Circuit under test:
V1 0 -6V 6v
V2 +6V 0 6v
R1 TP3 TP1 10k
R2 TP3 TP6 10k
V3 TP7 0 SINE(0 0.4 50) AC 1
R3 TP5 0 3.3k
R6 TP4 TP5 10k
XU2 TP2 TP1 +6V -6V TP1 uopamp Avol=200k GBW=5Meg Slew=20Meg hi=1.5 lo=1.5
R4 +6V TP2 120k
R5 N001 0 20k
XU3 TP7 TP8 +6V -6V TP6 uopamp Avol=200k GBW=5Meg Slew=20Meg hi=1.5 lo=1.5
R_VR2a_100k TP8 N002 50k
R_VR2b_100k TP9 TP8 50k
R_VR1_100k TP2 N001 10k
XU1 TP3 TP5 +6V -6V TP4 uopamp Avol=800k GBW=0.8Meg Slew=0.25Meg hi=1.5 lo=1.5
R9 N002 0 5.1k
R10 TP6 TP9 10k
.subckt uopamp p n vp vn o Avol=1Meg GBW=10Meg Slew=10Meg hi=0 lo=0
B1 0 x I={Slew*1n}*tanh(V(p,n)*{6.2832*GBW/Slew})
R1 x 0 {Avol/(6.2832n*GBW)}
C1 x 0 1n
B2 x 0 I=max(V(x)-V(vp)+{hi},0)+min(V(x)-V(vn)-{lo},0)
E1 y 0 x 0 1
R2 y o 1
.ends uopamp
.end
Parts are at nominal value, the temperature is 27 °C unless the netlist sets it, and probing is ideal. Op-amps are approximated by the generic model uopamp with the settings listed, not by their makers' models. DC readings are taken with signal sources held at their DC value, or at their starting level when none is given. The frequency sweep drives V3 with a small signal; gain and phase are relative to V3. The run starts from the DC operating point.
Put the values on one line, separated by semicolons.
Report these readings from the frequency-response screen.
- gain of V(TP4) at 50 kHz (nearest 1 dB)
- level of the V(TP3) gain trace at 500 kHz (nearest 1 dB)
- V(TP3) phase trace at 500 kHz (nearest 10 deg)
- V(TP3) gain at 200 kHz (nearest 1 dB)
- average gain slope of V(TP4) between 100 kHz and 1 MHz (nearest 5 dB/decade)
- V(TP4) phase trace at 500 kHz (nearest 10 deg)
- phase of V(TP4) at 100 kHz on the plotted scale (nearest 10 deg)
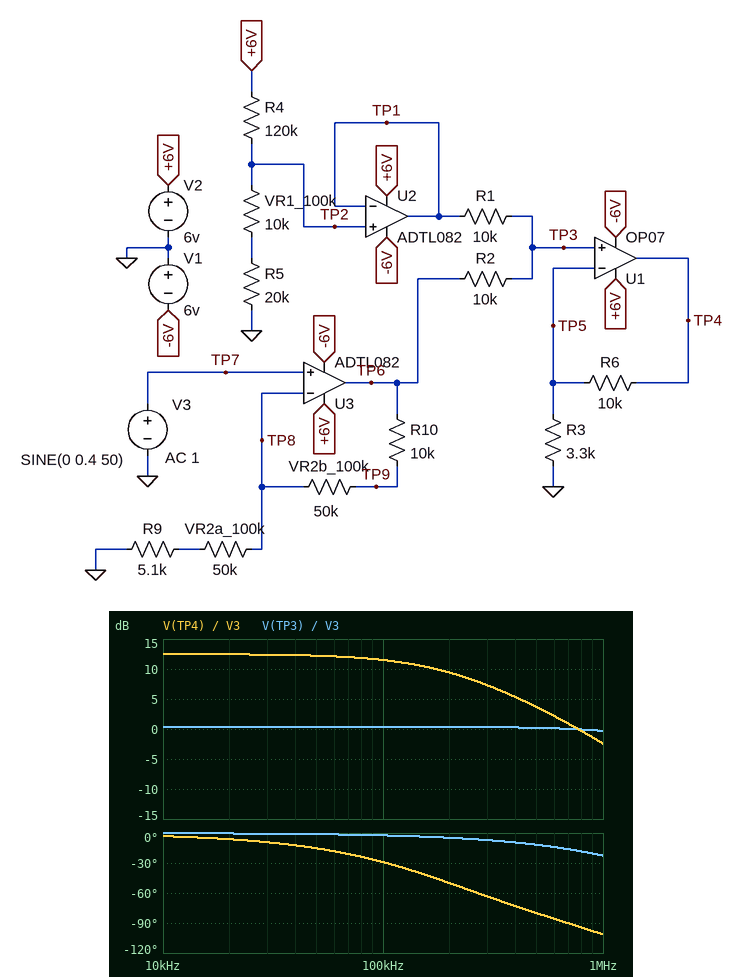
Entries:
12 dB; 0 dB; -10 deg; 0 dB; -15 dB/decade; -80 deg; -30 deg
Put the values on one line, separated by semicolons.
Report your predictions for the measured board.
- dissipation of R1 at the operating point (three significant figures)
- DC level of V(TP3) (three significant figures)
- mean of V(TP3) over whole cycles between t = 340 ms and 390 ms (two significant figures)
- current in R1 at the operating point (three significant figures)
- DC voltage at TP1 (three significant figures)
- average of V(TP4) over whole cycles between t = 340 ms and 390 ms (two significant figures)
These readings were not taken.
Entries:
36.0 µW; 600 mV; 600 mV; 60.0 µA; 1.20 V; 2.4 V
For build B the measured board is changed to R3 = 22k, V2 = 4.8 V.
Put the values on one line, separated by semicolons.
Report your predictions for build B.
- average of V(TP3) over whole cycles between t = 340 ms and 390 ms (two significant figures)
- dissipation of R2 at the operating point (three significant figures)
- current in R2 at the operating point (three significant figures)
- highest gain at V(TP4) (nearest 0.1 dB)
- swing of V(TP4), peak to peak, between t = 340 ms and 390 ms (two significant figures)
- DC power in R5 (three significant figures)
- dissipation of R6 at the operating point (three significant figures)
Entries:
480 mV; 23.0 µW; 48.0 µA; 3.6 dB; 1.2 V; 20.5 µW; 4.76 µW
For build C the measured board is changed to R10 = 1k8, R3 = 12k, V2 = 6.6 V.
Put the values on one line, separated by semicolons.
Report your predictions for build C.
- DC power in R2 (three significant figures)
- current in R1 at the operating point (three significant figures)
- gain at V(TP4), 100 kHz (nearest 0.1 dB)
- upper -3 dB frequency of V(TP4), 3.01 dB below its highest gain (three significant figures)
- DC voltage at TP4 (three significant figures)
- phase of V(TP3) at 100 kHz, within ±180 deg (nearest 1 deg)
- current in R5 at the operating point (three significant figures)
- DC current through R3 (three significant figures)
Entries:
43.6 µW; 66.0 µA; 4.8 dB; 425 kHz; 1.21 V; -2 deg; 44.0 µA; 55.0 µA
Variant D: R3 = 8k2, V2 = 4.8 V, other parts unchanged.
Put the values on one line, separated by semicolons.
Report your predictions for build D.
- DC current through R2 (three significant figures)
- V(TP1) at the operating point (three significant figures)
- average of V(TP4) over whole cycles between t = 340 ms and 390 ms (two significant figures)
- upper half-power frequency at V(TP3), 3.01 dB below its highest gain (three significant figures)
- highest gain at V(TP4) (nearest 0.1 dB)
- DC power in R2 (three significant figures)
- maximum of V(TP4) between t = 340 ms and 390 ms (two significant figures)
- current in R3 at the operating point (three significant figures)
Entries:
48.0 µA; 960 mV; 1.1 V; 2.39 MHz; 7.3 dB; 23.0 µW; 2.0 V; 58.5 µA
